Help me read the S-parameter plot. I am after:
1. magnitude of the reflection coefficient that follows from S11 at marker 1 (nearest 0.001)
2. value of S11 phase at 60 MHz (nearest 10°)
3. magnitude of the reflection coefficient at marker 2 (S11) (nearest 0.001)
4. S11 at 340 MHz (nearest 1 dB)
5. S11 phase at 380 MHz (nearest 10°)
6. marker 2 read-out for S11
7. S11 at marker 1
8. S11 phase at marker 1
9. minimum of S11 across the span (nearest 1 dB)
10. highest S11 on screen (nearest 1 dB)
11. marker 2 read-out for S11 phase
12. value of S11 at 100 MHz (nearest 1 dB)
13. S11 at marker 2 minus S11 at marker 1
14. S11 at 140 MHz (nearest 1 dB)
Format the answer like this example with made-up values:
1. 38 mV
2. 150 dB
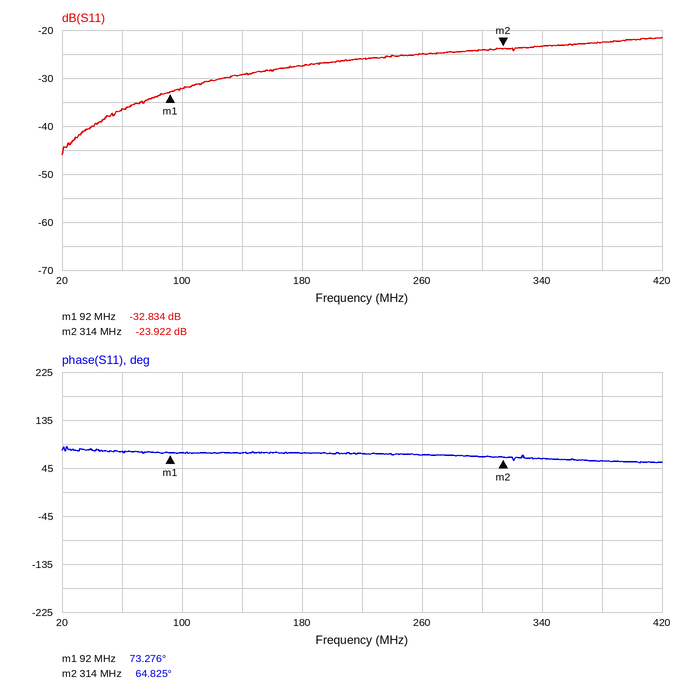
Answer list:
1. 0.023
2. 80°
3. 0.064
4. -23 dB
5. 60°
6. -23.922 dB
7. -32.834 dB
8. 73.276°
9. -46 dB
10. -22 dB
11. 64.825°
12. -32 dB
13. 8.912 dB
14. -29 dB
